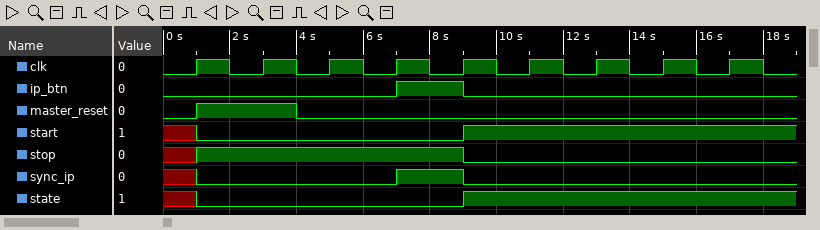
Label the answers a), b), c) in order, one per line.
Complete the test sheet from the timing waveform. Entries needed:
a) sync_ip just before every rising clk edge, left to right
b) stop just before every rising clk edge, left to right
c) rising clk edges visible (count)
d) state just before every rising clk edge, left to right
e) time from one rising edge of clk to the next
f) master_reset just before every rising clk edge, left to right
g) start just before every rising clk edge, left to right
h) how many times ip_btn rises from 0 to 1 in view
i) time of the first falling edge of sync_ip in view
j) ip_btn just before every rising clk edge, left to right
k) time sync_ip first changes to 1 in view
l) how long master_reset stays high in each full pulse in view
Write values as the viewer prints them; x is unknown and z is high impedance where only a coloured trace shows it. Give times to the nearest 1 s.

a) x 0 0 0 1 0 0 0 0
b) x 1 1 1 1 0 0 0 0
c) 9
d) x 0 0 0 0 1 1 1 1
e) 2 s
f) 0 1 0 0 0 0 0 0 0
g) x 0 0 0 0 1 1 1 1
h) 1
i) 9 s
j) 0 0 0 0 1 0 0 0 0
k) 7 s
l) 3 s
